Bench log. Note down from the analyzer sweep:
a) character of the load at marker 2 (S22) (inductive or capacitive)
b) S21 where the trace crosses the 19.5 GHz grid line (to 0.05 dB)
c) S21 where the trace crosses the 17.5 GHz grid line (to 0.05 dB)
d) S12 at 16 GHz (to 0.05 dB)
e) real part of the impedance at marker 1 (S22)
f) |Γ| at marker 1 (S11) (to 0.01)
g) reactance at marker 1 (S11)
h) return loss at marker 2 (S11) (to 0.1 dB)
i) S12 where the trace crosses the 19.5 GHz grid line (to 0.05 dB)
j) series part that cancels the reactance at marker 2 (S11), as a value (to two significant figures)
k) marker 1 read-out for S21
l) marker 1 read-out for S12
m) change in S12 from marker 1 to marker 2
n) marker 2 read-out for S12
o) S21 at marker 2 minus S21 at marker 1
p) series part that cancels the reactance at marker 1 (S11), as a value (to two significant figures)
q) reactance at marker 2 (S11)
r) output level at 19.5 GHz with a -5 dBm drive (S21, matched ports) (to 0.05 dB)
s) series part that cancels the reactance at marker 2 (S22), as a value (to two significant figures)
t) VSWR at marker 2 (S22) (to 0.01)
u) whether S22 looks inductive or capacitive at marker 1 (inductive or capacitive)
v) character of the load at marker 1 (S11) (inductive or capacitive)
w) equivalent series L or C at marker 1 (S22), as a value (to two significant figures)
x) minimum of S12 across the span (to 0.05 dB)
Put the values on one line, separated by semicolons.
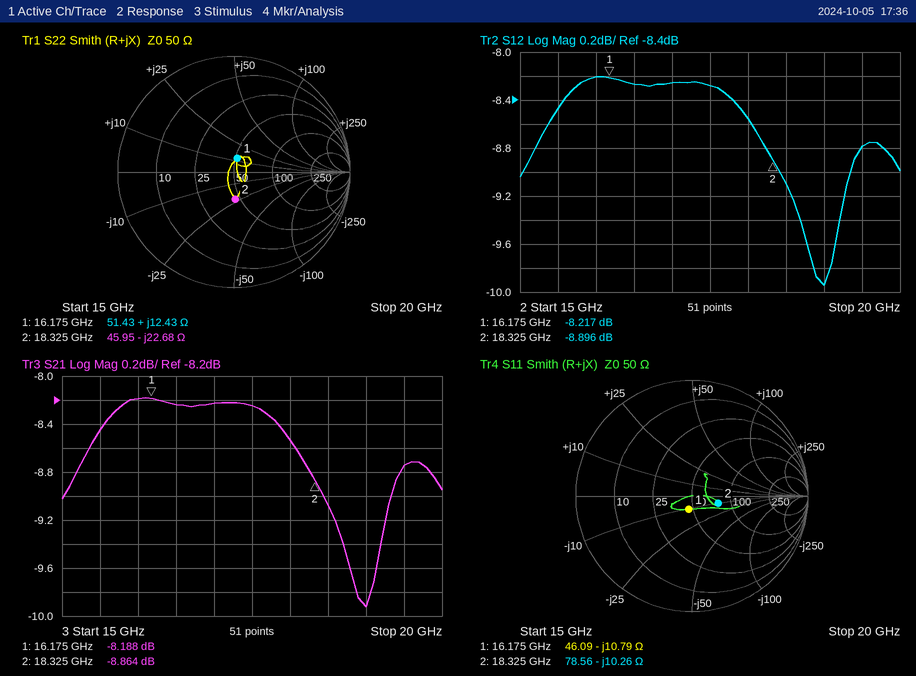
capacitive; -8.75 dB; -8.25 dB; -8.20 dB; 51.43 Ω; 0.12; -10.79 Ω; 12.6 dB; -8.80 dB; 89 pH; -8.188 dB; -8.217 dB; -0.679 dB; -8.896 dB; -0.676 dB; 110 pH; -10.26 Ω; -13.75 dBm; 200 pH; 1.61; inductive; capacitive; 120 pH; -9.95 dB
